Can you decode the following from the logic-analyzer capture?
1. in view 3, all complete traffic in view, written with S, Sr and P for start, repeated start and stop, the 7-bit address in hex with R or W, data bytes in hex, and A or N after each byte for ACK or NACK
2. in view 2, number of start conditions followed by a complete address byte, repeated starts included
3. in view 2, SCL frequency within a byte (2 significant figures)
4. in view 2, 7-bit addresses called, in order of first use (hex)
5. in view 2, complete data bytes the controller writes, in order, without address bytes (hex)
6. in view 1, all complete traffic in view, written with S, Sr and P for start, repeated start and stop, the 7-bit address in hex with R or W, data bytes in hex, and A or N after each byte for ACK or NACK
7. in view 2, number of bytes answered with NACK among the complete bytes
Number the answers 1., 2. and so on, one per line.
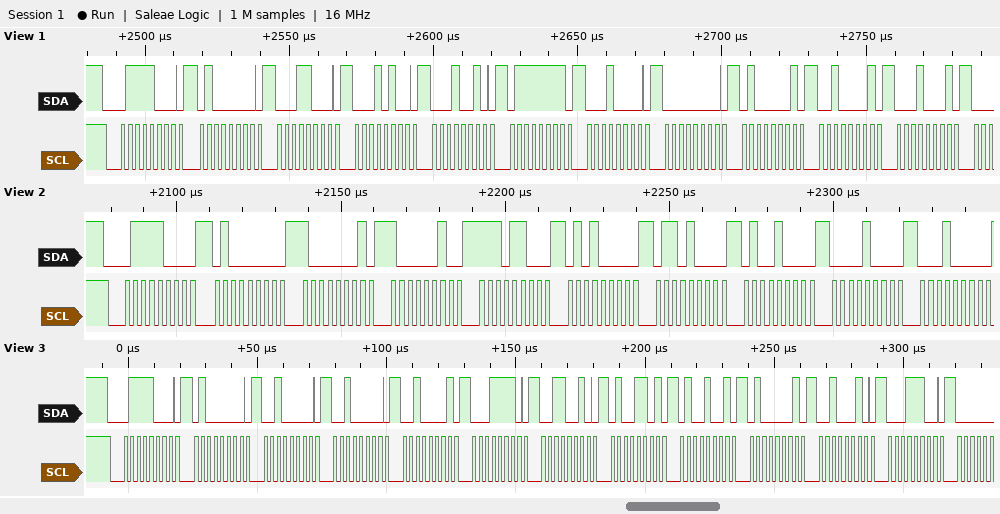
1. S 3CW A 40 A 20 A 20 A 21 A 1E A 32 A 4D A 49 A 41 A 22 A 1C A
2. 1
3. 400 kHz
4. 0x3C
5. 40 81 82 EC 50 68 48 08 10
6. S 3CW A 40 A 18 A 14 A 12 A 7F A 10 A 00 A 41 A 21 A 11 A
7. 0
